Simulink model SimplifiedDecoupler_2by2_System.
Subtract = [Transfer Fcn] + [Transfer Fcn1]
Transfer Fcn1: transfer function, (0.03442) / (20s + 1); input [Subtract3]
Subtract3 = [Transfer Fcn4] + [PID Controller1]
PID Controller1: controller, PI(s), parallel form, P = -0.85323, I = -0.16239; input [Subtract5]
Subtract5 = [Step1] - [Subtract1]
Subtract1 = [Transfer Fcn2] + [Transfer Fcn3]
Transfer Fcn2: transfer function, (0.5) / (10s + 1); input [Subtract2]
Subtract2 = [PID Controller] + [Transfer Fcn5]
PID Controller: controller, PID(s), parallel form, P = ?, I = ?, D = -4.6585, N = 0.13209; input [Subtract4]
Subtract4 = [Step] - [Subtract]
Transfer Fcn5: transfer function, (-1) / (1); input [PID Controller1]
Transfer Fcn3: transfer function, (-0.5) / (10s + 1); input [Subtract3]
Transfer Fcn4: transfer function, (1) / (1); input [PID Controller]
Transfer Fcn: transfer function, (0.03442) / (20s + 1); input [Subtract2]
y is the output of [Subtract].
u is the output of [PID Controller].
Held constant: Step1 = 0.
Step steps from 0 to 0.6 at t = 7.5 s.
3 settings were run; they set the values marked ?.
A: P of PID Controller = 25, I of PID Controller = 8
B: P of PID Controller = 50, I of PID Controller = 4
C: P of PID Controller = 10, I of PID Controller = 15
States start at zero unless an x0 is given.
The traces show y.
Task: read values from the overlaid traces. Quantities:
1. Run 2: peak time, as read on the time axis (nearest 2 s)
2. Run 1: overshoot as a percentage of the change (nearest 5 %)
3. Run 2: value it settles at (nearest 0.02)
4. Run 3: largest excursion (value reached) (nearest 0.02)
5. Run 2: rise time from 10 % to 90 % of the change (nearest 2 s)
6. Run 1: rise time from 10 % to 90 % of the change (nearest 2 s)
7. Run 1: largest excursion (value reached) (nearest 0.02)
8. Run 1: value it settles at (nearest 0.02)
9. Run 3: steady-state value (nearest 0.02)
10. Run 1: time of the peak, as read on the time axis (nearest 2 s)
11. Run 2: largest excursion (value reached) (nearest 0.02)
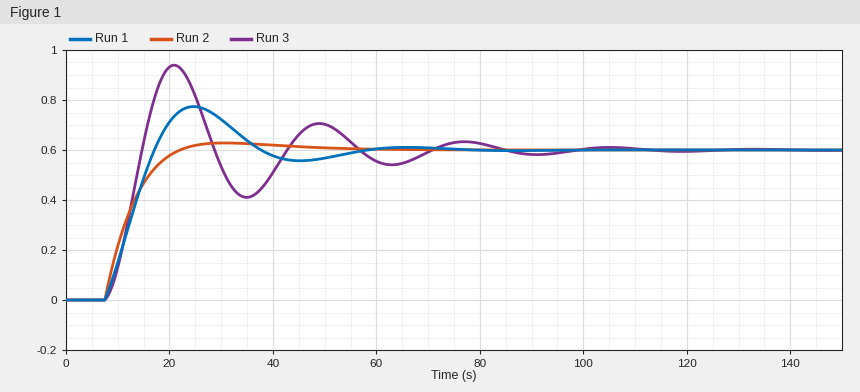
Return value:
30 s
30 %
0.60
0.94
10 s
8 s
0.78
0.60
0.60
24 s
0.62
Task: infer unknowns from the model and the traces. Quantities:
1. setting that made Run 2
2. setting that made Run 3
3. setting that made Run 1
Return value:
B
C
A
